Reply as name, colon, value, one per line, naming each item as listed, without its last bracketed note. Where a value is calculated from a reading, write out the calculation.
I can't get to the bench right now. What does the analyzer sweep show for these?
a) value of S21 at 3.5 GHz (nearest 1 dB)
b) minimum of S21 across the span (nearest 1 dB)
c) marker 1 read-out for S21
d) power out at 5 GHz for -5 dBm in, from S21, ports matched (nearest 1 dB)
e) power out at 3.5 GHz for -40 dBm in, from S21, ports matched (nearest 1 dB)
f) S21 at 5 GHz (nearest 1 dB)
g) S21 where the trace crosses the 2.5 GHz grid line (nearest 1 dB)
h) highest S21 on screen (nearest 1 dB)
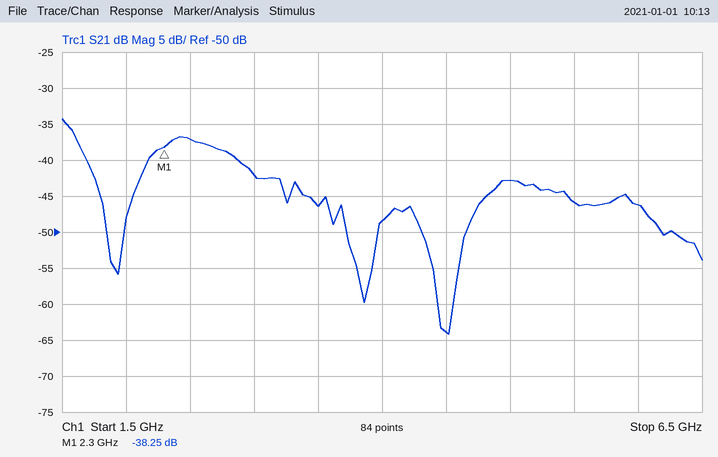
value of S21 at 3.5 GHz: -46 dB
minimum of S21 across the span: -64 dB
marker 1 read-out for S21: -38.25 dB
power out at 5 GHz for -5 dBm in, from S21, ports matched: -5 dBm + (-43 dB) = -48 dBm
power out at 3.5 GHz for -40 dBm in, from S21, ports matched: -40 dBm + (-46 dB) = -86 dBm
S21 at 5 GHz: -43 dB
S21 where the trace crosses the 2.5 GHz grid line: -37 dB
highest S21 on screen: -34 dB
